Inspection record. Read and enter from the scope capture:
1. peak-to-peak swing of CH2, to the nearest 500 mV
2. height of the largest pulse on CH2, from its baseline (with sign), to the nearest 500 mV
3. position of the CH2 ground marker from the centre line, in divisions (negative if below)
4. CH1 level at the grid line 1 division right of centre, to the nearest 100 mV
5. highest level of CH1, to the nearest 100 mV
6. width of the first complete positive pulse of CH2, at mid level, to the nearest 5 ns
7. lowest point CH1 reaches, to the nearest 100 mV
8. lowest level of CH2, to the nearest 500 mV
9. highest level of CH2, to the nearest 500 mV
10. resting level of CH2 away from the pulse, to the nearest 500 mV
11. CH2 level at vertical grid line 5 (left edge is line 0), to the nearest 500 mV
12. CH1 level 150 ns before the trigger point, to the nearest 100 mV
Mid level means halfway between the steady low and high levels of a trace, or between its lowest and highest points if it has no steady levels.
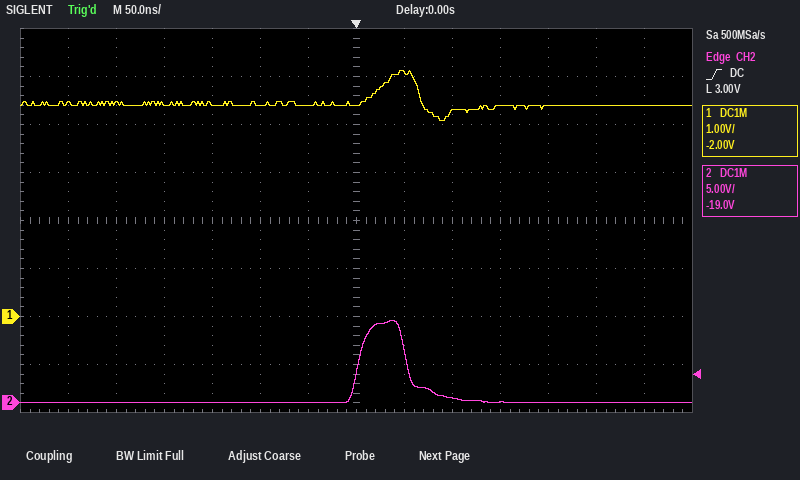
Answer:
8.5 V
+8.5 V
-3.8 div
5.1 V
5.1 V
50 ns
4.1 V
0.0 V
8.5 V
0.0 V
0.0 V
4.4 V
